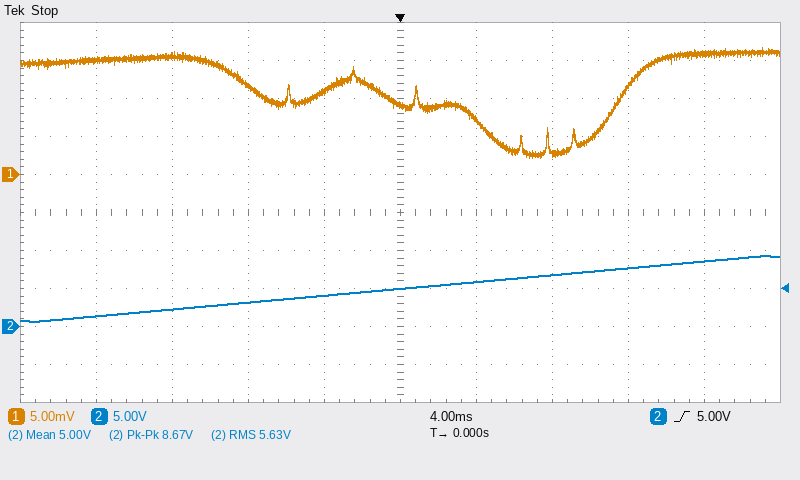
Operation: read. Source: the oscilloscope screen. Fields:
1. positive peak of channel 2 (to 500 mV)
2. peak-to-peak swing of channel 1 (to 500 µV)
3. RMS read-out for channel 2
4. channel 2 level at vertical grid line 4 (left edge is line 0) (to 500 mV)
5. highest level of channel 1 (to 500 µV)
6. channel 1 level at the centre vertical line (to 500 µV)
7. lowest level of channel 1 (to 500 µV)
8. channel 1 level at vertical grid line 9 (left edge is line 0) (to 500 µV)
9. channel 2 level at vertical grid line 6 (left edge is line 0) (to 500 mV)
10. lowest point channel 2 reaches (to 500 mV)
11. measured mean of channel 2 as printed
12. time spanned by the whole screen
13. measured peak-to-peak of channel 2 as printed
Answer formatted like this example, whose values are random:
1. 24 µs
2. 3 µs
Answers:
1. 9.5 V
2. 14.5 mV
3. 5.63 V
4. 4.0 V
5. 16.5 mV
6. 9.0 mV
7. 2.0 mV
8. 16.0 mV
9. 6.0 V
10. 500 mV
11. 5.00 V
12. 40 ms
13. 8.67 V
